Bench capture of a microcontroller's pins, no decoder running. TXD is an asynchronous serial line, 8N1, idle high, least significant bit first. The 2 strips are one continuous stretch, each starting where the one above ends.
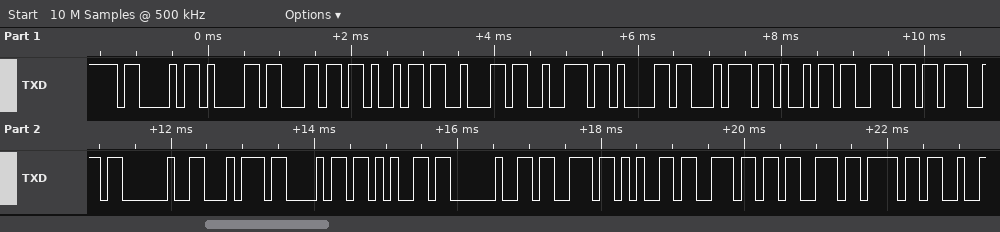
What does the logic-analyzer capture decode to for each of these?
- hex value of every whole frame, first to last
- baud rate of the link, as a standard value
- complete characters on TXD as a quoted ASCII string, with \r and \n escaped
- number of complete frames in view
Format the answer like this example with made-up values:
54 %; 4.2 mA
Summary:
43 61 6C 69 62 72 61 74 69 6E 67 20 74 68 65 20 73 65 6E 73 6F; 9600 baud; "Calibrating the senso"; 21
